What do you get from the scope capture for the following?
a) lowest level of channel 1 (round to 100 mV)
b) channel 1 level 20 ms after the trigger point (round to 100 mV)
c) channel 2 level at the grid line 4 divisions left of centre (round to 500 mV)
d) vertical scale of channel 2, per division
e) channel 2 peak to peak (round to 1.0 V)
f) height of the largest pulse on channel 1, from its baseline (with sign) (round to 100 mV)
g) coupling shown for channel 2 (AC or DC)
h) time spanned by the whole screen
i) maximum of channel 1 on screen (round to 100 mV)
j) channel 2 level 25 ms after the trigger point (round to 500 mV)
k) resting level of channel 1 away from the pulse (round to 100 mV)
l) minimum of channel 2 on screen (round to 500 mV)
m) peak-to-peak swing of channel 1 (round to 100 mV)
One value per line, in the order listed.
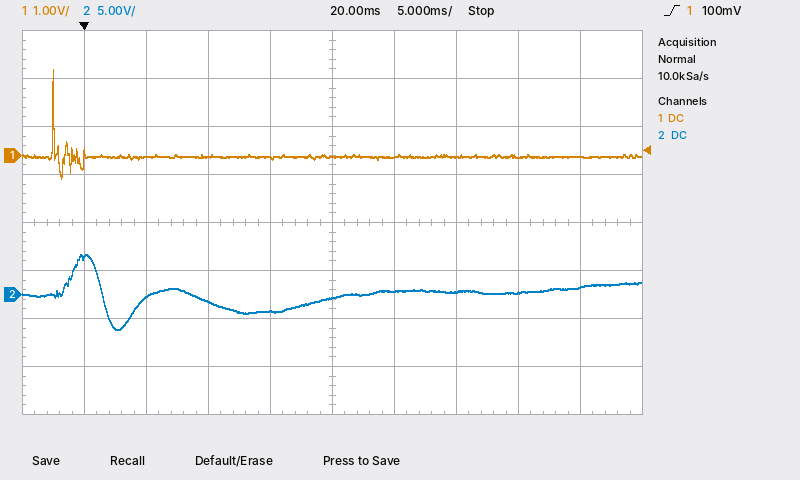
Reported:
-500 mV
0.0 V
4.0 V
5 V
8.0 V
+1.8 V
DC
50 ms
1.8 V
500 mV
0.0 V
-3.5 V
2.3 V
